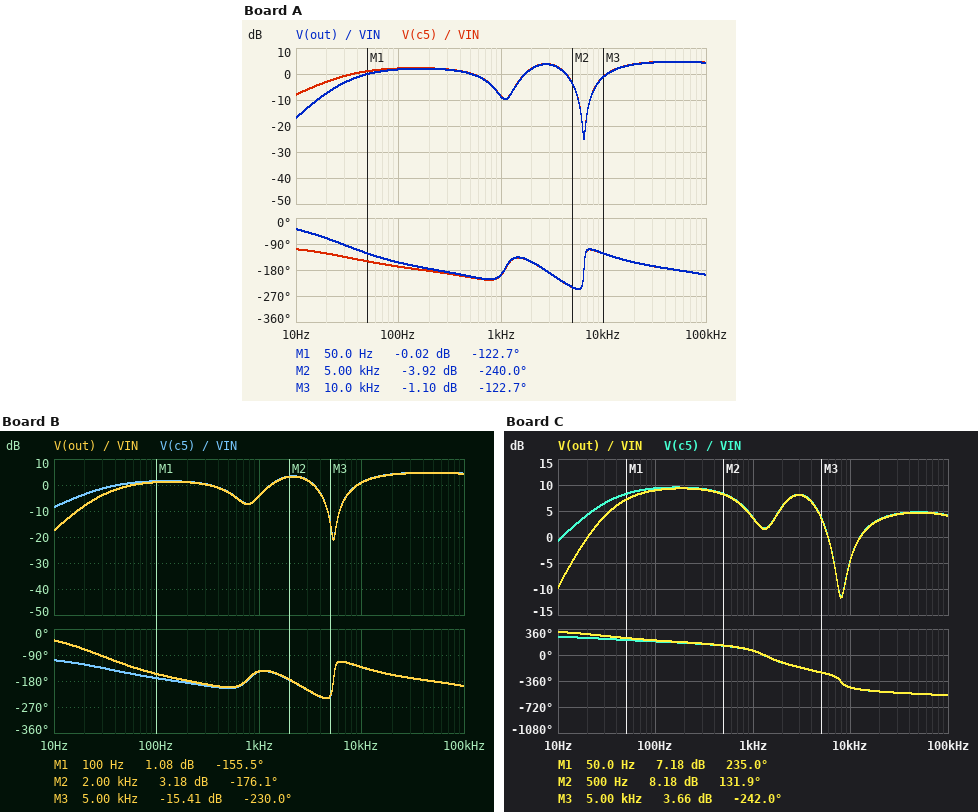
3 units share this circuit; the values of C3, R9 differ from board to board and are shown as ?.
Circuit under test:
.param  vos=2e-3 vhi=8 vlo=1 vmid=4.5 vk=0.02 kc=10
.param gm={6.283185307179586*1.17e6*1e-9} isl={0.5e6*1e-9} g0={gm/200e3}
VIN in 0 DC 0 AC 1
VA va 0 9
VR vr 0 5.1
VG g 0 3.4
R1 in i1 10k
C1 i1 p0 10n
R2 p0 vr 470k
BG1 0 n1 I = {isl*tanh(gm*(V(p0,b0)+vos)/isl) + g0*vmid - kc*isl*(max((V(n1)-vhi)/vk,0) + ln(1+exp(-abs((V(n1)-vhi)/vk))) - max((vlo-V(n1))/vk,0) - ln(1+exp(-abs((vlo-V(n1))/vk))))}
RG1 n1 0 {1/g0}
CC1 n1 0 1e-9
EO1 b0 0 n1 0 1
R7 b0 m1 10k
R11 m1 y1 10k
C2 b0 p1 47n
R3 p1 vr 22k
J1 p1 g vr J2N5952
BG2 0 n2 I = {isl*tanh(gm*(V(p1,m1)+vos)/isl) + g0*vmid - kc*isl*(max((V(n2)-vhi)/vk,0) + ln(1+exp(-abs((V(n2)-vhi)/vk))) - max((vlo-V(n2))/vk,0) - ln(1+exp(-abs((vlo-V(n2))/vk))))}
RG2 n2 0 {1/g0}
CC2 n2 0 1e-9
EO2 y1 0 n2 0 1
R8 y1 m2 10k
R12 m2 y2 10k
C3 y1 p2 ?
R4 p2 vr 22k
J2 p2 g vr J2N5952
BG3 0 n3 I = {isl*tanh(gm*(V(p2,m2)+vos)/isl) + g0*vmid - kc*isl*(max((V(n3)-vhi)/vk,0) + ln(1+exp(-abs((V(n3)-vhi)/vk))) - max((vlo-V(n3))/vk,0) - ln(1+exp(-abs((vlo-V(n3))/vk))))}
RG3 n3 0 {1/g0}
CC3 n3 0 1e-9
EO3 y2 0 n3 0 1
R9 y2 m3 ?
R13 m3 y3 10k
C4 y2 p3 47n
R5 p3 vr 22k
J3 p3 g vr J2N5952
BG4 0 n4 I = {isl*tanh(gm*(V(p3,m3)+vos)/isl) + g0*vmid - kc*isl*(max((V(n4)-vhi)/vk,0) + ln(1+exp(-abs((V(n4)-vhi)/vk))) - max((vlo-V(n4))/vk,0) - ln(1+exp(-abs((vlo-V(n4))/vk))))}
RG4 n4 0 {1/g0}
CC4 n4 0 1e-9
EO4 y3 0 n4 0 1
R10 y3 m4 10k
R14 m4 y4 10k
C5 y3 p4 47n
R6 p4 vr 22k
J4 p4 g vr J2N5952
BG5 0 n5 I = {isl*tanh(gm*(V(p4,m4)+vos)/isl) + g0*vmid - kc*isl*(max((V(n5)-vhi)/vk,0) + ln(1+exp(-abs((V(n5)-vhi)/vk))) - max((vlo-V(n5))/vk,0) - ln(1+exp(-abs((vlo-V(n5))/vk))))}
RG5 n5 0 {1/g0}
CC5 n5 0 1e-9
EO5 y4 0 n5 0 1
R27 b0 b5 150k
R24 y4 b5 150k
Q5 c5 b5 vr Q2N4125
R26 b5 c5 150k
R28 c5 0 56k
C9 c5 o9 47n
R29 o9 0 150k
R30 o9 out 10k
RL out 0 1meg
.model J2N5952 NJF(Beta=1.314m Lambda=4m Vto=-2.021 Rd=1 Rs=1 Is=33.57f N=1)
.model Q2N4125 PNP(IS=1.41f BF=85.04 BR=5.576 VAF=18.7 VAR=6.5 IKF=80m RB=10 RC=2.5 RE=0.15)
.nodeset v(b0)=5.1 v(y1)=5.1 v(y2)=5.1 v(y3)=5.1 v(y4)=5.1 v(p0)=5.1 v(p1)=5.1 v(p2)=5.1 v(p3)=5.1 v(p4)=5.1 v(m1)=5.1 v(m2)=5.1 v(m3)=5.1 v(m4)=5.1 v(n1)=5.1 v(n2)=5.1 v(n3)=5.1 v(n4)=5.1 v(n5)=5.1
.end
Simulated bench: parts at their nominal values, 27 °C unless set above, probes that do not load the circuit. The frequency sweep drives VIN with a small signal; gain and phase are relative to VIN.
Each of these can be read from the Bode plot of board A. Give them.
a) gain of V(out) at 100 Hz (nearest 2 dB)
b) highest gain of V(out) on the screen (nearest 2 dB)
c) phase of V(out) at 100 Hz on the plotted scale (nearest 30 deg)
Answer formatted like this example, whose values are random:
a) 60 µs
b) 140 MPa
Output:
a) 2 dB
b) 4 dB
c) -150 deg
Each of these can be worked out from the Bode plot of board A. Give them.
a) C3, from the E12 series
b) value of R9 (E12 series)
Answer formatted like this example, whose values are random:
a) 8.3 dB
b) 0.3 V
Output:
a) 56 nF
b) 18 kΩ
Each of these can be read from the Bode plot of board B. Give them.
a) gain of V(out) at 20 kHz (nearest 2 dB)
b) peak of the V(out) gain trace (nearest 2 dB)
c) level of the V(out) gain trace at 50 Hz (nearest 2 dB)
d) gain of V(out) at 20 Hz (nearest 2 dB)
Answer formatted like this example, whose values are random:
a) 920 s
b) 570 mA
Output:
a) 4 dB
b) 4 dB
c) 0 dB
d) -8 dB
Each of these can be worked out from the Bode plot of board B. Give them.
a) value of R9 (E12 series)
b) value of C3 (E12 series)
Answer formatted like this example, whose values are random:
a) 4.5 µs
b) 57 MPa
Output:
a) 22 kΩ
b) 150 nF
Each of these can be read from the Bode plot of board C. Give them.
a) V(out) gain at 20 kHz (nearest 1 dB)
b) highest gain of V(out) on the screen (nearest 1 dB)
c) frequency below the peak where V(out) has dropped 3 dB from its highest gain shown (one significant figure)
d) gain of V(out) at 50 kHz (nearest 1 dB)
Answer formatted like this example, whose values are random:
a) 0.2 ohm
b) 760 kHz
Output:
a) 3 dB
b) 9 dB
c) 40 Hz
d) 5 dB
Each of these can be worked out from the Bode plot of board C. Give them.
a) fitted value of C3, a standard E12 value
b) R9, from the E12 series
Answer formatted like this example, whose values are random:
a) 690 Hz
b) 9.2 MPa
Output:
a) 56 nF
b) 3.9 kΩ
